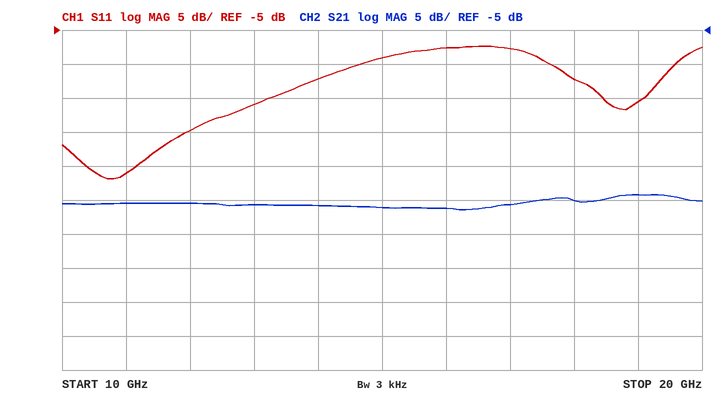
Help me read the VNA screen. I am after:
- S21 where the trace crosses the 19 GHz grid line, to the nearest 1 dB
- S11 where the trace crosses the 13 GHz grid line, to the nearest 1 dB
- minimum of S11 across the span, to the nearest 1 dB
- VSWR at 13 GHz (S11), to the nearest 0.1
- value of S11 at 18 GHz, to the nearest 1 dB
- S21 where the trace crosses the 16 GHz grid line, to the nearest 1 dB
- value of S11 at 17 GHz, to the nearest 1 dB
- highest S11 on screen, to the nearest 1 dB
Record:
-29 dB
-16 dB
-27 dB
1.4
-12 dB
-31 dB
-8 dB
-7 dB
